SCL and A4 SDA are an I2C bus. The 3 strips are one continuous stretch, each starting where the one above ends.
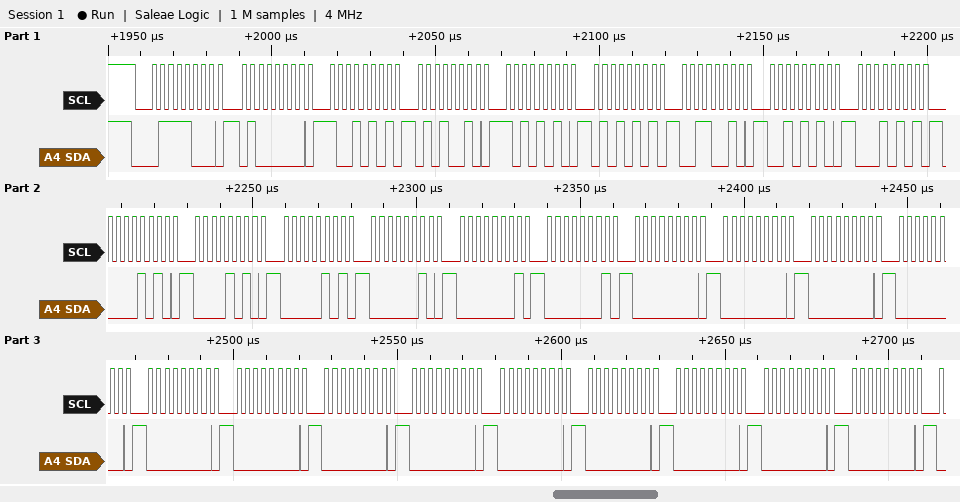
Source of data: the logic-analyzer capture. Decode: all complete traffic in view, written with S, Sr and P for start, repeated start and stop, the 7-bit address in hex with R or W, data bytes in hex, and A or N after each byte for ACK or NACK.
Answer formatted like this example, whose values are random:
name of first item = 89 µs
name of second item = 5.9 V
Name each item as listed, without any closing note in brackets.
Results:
all complete traffic in view, written with S, Sr and P for start, repeated start and stop, the 7-bit address in hex with R or W, data bytes in hex, and A or N after each byte for ACK or NACK = S 3CW A 40 A 95 A 52 A AA A 55 A 32 A 2A A 15 A 0A A 0A A 05 A 02 A 01 A 01 A 00 A 00 A 00 A 00 A 00 A 00 A 00 A 00 A 00 A 00 A 00 A 00 A 00 A
